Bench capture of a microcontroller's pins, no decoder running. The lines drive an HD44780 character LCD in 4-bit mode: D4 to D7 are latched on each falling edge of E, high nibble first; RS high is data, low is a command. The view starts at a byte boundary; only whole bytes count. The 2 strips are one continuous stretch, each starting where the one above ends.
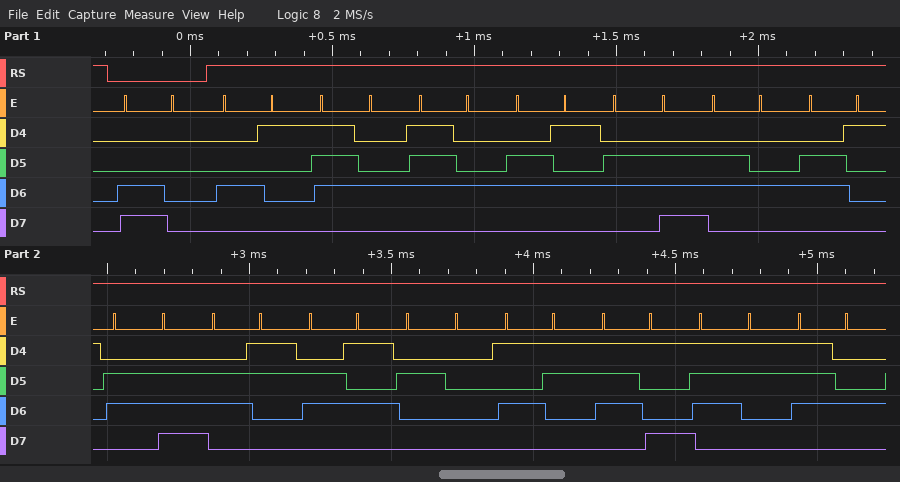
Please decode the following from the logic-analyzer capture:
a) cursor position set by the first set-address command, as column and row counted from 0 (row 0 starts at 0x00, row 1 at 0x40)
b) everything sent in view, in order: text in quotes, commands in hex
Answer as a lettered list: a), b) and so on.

a) column 0, row 1
b) 0xC0 "Attendance Syst"
